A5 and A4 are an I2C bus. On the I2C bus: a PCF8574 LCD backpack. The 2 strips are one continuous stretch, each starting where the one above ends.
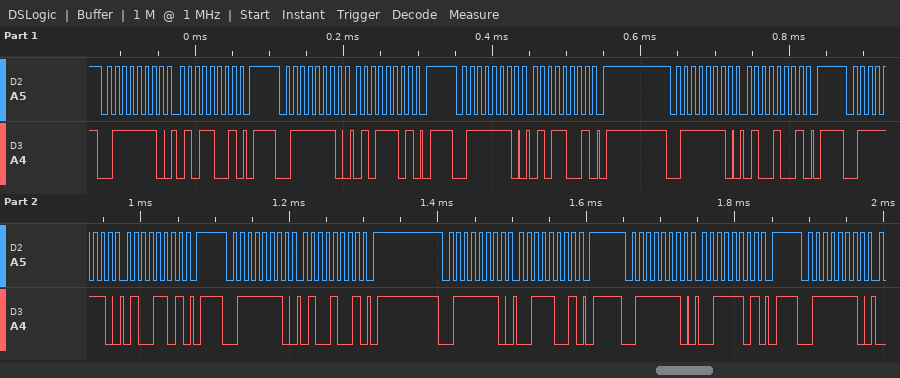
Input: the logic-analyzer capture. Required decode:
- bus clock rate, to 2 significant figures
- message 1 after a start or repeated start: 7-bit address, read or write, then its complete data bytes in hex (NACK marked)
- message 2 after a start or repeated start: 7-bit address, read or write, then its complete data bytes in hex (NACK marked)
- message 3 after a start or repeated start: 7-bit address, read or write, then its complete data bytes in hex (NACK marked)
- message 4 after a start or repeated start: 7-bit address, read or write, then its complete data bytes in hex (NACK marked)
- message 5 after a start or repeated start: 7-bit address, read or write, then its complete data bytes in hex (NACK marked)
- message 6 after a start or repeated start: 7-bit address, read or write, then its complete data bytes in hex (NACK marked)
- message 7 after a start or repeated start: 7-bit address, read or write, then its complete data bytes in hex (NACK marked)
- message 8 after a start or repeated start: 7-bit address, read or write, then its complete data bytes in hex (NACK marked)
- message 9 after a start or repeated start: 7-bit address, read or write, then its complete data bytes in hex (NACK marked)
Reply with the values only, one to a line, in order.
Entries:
100 kHz
0x3F write: 59
0x3F write: 5D
0x3F write: 59
0x3F write: 49
0x3F write: 4D
0x3F write: 49
0x3F write: 39
0x3F write: 3D
0x3F write
